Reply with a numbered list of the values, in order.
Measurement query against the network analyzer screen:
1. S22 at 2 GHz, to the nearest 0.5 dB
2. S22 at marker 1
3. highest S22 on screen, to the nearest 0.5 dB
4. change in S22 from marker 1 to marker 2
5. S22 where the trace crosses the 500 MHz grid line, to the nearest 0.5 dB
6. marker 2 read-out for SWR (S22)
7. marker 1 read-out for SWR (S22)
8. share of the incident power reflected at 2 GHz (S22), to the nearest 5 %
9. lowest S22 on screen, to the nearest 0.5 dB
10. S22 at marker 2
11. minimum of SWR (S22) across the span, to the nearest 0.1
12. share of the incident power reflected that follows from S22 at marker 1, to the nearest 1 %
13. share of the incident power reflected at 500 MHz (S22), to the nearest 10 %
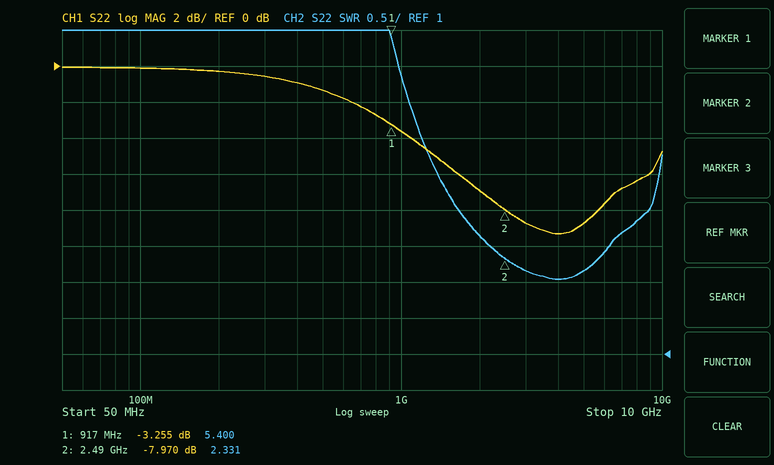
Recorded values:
1. -7.0 dB
2. -3.255 dB
3. 0.0 dB
4. -4.715 dB
5. -1.5 dB
6. 2.331
7. 5.400
8. 20 %
9. -9.5 dB
10. -7.970 dB
11. 2.0
12. 47 %
13. 70 %
